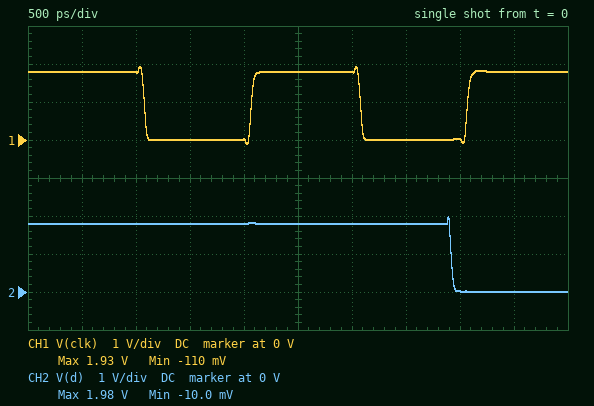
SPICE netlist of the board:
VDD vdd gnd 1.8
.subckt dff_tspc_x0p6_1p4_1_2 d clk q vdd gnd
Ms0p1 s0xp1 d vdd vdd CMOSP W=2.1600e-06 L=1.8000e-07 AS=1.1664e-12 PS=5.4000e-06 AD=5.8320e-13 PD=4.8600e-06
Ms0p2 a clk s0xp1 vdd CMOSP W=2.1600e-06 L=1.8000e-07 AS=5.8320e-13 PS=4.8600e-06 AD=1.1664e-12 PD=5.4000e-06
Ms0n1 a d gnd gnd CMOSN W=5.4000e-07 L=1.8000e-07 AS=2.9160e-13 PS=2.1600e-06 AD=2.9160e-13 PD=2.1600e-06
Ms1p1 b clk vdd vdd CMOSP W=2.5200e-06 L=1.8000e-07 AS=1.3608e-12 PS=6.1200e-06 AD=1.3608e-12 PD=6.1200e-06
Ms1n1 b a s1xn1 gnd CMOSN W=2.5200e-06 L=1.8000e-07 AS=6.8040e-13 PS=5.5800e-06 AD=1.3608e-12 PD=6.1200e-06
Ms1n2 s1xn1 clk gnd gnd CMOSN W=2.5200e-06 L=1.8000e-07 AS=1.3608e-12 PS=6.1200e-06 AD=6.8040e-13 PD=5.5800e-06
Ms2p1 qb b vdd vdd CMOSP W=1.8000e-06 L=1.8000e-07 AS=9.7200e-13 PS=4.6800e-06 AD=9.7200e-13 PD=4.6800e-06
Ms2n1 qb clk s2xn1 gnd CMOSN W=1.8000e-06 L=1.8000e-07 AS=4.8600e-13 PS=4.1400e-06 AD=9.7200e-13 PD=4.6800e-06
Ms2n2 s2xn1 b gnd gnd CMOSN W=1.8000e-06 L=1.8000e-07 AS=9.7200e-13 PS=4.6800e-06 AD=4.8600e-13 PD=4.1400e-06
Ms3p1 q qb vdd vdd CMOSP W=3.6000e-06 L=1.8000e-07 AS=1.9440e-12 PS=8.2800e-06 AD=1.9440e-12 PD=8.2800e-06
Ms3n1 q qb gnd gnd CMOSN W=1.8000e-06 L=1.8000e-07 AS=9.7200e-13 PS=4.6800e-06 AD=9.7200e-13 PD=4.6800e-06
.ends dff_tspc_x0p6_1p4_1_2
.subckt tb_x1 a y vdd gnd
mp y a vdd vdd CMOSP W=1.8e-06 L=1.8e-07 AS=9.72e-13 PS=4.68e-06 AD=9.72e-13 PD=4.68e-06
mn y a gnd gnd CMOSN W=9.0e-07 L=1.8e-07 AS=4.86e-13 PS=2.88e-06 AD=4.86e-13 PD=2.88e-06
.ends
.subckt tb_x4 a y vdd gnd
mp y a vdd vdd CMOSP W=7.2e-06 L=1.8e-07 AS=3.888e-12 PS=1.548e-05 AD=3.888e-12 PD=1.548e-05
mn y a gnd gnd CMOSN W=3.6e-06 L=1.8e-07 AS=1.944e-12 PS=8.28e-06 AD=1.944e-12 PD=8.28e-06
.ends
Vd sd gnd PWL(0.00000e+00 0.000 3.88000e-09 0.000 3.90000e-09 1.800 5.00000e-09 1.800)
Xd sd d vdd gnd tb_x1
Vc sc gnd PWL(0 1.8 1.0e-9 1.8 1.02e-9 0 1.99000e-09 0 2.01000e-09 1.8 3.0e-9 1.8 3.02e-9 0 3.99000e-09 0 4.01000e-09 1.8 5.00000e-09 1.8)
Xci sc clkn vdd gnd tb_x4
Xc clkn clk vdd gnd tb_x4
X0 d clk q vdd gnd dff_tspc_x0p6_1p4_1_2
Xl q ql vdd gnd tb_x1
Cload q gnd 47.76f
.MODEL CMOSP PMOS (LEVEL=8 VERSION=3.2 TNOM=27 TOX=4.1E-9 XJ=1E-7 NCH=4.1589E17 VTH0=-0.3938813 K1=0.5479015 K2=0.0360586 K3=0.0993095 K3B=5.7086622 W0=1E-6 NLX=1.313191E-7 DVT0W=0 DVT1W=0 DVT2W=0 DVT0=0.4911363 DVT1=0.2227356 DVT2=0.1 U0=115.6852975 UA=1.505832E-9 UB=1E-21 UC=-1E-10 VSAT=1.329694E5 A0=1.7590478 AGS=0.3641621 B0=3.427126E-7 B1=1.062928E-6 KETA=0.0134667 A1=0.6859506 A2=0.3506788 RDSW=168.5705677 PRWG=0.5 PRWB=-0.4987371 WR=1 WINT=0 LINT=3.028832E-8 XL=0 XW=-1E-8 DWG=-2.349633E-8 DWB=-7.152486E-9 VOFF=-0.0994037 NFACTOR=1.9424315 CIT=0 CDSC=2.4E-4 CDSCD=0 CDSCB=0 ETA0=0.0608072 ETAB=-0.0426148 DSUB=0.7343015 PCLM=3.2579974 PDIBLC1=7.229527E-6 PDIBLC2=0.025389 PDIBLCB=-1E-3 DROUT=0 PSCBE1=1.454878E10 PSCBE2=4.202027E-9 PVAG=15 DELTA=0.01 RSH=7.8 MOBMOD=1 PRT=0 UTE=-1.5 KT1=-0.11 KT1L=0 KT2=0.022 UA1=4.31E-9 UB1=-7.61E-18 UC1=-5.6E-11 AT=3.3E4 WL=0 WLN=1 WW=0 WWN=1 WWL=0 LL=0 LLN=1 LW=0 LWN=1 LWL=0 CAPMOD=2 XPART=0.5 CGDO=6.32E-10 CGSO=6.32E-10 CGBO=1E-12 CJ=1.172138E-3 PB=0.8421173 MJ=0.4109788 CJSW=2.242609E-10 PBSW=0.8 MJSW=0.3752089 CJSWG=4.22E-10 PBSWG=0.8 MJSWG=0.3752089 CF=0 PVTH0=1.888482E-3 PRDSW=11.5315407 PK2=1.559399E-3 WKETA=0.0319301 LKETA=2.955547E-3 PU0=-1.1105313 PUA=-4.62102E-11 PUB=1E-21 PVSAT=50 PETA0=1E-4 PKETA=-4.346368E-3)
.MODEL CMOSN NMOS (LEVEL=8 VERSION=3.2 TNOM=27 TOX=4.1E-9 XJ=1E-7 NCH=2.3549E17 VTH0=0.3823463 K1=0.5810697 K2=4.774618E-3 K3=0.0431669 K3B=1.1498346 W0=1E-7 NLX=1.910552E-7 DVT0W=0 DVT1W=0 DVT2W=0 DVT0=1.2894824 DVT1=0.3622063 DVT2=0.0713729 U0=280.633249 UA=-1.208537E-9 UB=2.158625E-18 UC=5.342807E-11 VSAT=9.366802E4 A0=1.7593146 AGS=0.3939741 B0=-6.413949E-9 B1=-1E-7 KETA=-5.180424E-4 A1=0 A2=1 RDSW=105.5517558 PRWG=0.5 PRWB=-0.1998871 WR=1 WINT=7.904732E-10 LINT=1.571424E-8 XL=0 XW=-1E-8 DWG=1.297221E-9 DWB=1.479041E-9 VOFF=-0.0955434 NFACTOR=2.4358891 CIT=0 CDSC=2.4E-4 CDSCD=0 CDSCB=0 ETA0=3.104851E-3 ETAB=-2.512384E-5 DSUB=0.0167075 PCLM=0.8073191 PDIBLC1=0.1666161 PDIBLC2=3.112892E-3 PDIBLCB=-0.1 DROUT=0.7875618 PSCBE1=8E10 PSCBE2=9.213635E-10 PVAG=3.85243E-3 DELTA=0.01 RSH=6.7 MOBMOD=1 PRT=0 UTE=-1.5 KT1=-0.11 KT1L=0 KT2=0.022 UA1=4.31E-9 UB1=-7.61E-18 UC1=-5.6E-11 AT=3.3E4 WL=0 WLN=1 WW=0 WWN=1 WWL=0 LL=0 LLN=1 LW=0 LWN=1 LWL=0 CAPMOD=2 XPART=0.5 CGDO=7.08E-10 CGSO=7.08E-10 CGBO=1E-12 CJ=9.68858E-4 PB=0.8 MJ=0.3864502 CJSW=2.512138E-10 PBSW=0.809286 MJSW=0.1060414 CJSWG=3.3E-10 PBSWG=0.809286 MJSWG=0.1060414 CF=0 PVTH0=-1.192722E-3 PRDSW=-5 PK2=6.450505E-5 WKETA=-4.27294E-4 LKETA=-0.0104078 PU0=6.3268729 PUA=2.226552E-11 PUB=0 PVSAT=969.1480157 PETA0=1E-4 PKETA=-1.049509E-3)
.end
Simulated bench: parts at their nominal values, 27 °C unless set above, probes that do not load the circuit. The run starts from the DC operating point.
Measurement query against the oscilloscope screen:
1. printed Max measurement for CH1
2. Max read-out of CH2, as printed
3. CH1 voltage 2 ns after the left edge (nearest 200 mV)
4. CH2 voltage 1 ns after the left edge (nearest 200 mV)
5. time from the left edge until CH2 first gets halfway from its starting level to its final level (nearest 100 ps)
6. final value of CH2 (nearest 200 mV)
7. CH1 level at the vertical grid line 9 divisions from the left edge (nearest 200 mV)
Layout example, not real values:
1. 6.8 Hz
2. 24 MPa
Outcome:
1. 1.93 V
2. 1.98 V
3. 0 V
4. 1.8 V
5. 3.9 ns
6. 0 V
7. 1.8 V
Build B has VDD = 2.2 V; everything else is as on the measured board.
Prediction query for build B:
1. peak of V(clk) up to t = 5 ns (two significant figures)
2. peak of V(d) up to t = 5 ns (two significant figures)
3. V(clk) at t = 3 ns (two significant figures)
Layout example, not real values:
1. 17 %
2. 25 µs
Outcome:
1. 2.3 V
2. 2.4 V
3. 2.2 V
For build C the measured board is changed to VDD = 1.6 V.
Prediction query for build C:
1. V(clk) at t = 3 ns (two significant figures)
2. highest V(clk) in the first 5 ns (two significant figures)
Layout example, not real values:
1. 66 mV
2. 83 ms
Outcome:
1. 1.6 V
2. 1.7 V
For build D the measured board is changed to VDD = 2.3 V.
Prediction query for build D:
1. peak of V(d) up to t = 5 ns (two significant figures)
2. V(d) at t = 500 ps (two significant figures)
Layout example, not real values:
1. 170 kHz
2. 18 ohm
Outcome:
1. 2.5 V
2. 2.3 V
